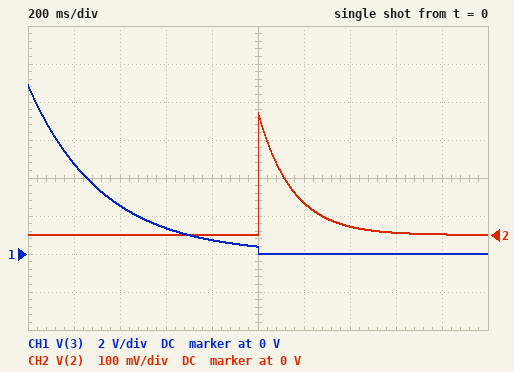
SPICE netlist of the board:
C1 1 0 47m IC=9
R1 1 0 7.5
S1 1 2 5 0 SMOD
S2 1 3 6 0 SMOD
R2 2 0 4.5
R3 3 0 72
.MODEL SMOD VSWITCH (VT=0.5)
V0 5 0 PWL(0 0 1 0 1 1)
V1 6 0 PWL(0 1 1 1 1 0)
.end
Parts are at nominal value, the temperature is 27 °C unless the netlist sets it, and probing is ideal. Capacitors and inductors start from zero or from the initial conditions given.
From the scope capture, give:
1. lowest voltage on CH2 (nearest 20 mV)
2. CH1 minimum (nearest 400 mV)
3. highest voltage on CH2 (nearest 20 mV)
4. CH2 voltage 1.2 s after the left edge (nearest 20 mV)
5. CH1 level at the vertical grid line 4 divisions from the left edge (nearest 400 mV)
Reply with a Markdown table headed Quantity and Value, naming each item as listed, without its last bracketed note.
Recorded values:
| Quantity | Value |
|---|---|
| lowest voltage on CH2 | 0 V |
| CH1 minimum | 0 V |
| highest voltage on CH2 | 320 mV |
| CH2 voltage 1.2 s after the left edge | 80 mV |
| CH1 level at the vertical grid line 4 divisions from the left edge | 800 mV |
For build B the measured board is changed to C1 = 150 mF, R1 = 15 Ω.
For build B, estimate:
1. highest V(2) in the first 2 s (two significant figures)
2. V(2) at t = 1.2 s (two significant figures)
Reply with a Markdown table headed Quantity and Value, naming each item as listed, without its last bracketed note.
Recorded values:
| Quantity | Value |
|---|---|
| highest V(2) in the first 2 s | 4.3 V |
| V(2) at t = 1.2 s | 3.1 V |
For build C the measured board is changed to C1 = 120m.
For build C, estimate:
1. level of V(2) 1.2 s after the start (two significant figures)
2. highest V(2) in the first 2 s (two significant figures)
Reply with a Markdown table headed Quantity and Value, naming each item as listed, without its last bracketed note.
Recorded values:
| Quantity | Value |
|---|---|
| level of V(2) 1.2 s after the start | 1.3 V |
| highest V(2) in the first 2 s | 2.2 V |
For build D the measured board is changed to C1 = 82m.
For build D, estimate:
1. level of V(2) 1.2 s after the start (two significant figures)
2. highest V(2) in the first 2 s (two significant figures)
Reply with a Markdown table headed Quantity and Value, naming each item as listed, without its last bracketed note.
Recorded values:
| Quantity | Value |
|---|---|
| level of V(2) 1.2 s after the start | 570 mV |
| highest V(2) in the first 2 s | 1.2 V |
